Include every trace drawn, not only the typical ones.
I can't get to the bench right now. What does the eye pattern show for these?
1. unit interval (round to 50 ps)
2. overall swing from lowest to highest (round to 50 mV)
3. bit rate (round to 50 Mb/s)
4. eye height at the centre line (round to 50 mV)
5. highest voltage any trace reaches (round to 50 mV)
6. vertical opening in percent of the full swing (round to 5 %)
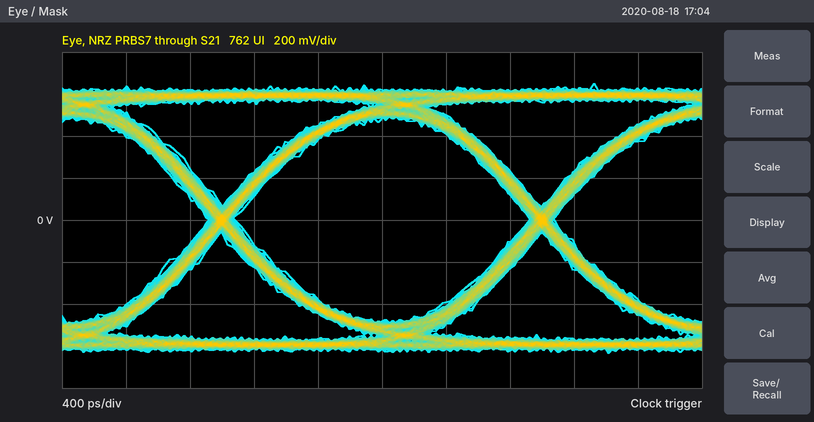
2.00 ns
1.30 V
500 Mb/s
950 mV
650 mV
75 %
